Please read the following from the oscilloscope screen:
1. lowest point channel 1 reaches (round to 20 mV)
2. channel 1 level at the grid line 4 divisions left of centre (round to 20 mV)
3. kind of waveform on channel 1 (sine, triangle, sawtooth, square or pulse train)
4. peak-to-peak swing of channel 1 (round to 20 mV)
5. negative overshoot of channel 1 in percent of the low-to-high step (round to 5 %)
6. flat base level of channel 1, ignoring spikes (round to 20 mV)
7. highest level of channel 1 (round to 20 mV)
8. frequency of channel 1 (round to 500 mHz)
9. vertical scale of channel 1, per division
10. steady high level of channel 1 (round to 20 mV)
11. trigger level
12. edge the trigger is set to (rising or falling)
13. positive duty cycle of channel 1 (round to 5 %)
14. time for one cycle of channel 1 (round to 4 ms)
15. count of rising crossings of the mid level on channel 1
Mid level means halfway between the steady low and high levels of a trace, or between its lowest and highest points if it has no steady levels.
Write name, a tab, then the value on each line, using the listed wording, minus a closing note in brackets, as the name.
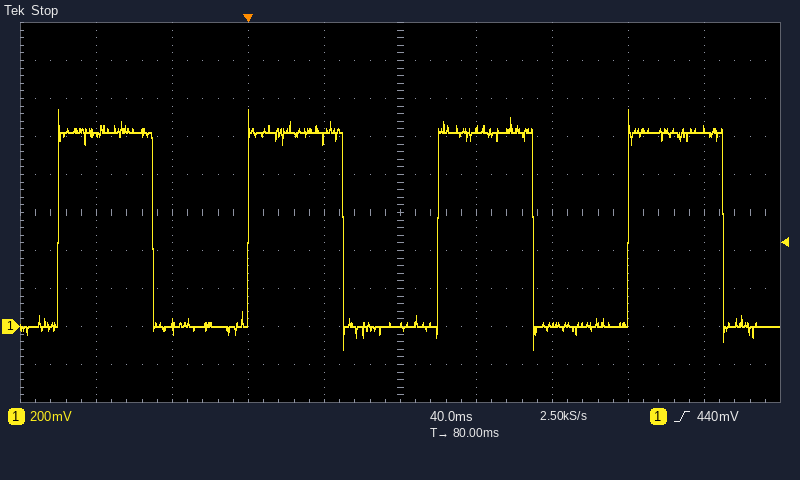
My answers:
lowest point channel 1 reaches	-120 mV
channel 1 level at the grid line 4 divisions left of centre	1.02 V
kind of waveform on channel 1	square
peak-to-peak swing of channel 1	1.26 V
negative overshoot of channel 1 in percent of the low-to-high step	10 %
flat base level of channel 1, ignoring spikes	0 mV
highest level of channel 1	1.14 V
frequency of channel 1	10.0 Hz
vertical scale of channel 1, per division	200 mV
steady high level of channel 1	1.02 V
trigger level	440 mV
edge the trigger is set to	rising
positive duty cycle of channel 1	50 %
time for one cycle of channel 1	100 ms
count of rising crossings of the mid level on channel 1	4
